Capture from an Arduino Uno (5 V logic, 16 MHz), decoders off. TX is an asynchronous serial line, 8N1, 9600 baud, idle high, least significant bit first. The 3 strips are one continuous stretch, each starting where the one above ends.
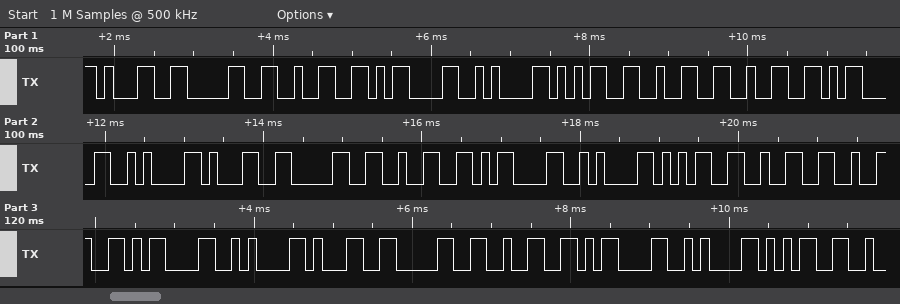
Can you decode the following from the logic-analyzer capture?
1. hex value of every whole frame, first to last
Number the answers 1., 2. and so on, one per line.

1. 31 30 32 0D 0A 35 32 32 0D 0A 31 30 32 0D 0A 35 32 32 0D 0A 31 30 32 0D 0A 35
